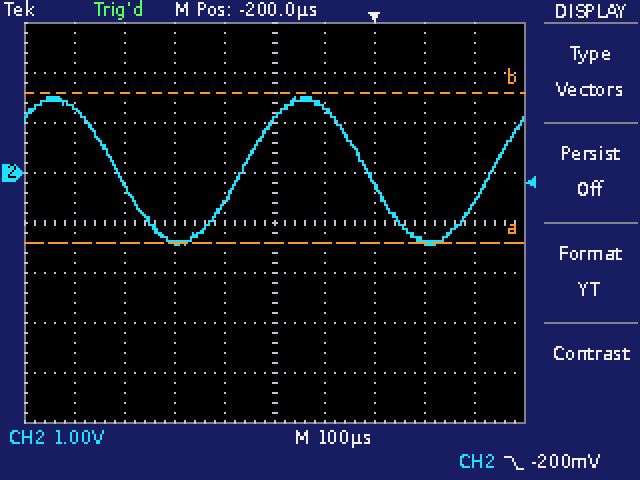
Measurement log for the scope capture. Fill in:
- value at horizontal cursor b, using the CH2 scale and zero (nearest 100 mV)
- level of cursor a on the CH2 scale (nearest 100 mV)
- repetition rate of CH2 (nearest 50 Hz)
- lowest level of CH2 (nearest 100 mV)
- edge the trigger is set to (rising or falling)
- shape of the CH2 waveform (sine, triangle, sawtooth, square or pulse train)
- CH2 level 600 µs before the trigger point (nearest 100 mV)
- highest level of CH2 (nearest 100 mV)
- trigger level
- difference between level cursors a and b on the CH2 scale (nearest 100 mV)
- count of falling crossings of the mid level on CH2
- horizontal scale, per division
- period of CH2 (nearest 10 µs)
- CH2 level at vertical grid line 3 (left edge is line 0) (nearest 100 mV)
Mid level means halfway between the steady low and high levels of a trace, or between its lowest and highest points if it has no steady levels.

1.6 V
-1.4 V
2.00 kHz
-1.4 V
falling
sine
1.3 V
1.5 V
-200 mV
3.0 V
2
100 µs
500 µs
-1.4 V
